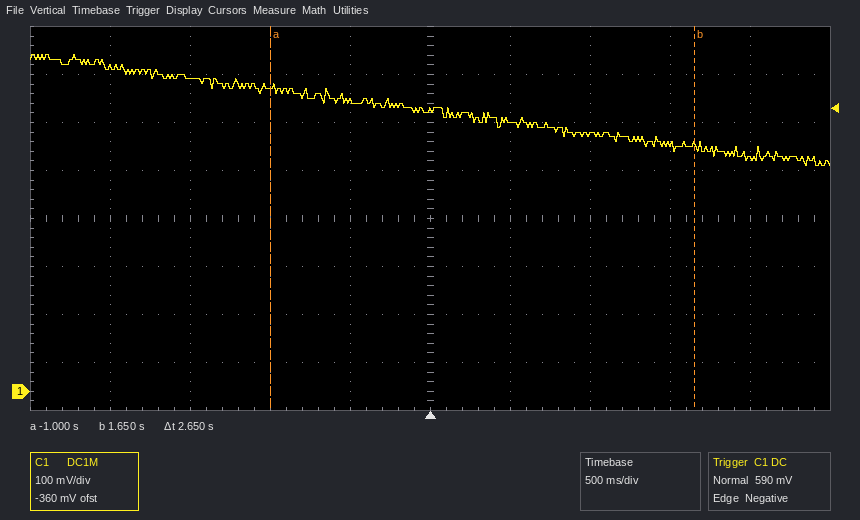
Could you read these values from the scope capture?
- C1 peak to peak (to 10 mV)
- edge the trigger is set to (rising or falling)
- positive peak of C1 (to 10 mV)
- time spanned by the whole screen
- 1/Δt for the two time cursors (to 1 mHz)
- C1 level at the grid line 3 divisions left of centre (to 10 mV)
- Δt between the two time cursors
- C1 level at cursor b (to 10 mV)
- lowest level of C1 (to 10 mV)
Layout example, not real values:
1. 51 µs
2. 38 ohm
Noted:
1. 230 mV
2. falling
3. 700 mV
4. 5 s
5. 377 mHz
6. 650 mV
7. 2.65 s
8. 510 mV
9. 470 mV
